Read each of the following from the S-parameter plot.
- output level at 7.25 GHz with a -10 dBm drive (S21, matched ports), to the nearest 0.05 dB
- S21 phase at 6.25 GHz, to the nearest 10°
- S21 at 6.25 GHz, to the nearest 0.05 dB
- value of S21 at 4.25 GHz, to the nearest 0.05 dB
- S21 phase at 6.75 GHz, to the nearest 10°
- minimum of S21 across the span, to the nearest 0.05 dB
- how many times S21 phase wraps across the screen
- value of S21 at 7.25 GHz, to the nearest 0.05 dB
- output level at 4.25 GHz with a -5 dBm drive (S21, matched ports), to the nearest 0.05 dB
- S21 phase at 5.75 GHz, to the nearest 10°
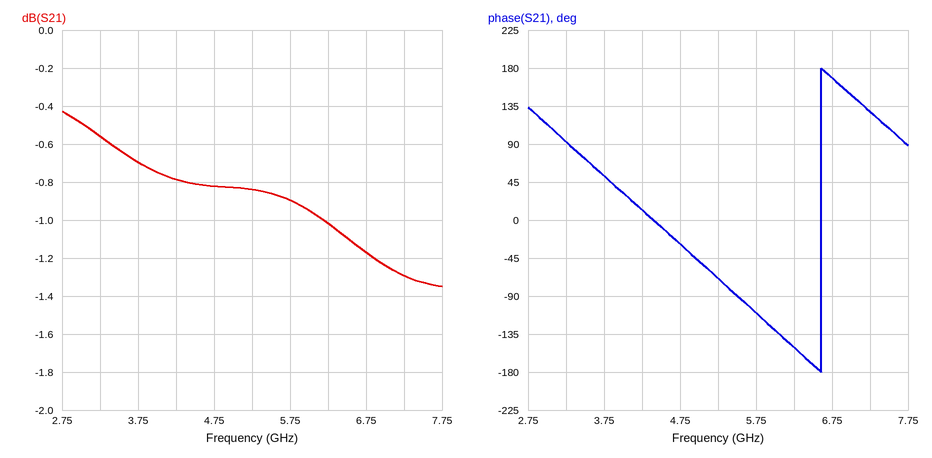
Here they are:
-11.30 dBm
-150°
-1.00 dB
-0.80 dB
170°
-1.35 dB
1
-1.30 dB
-5.80 dBm
-110°
